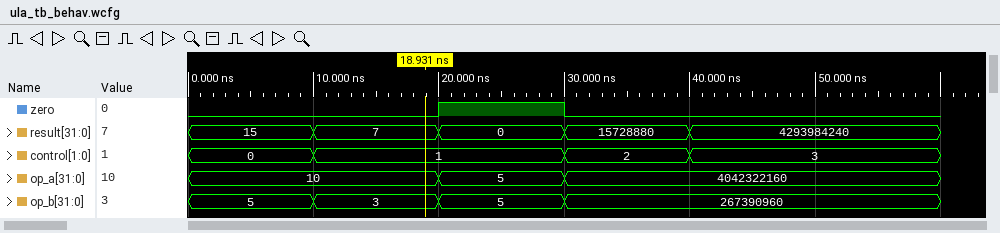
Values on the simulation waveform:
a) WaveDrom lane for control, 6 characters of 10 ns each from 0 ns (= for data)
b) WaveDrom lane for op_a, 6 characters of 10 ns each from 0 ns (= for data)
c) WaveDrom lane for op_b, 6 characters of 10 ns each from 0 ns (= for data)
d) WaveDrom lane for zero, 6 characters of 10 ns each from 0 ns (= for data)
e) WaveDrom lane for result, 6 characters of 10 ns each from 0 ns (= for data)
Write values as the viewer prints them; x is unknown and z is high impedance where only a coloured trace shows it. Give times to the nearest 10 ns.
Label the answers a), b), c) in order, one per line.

a) {name: 'control', wave: '==.==.', data: '0 1 2 3'}
b) {name: 'op_a', wave: '=.==..', data: '10 5 4042322160'}
c) {name: 'op_b', wave: '====..', data: '5 3 5 267390960'}
d) {name: 'zero', wave: '0.10..'}
e) {name: 'result', wave: '=====.', data: '15 7 0 15728880 4293984240'}
